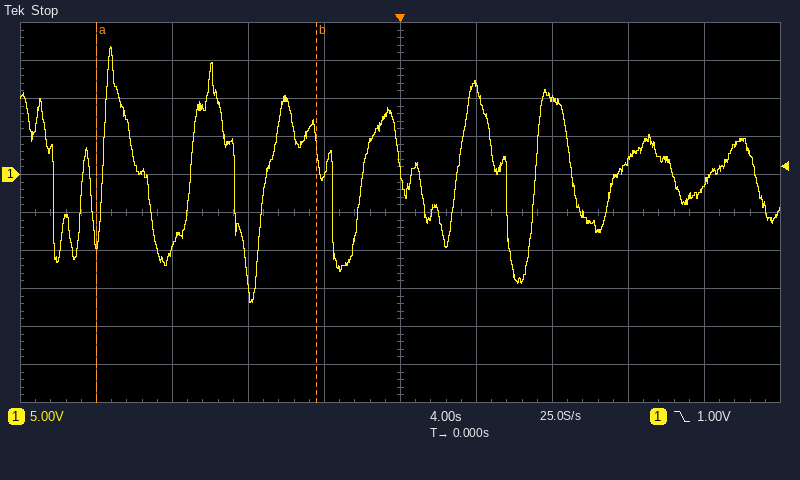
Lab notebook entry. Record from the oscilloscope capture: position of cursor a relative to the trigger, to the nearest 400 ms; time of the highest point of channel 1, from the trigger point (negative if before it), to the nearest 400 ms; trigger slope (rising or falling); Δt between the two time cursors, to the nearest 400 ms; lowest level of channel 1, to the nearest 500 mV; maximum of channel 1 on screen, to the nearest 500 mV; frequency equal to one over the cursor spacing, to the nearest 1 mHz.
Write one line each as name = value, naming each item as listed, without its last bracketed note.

position of cursor a relative to the trigger, to the nearest 400 ms = -16.0 s
time of the highest point of channel 1, from the trigger point (negative if before it), to the nearest 400 ms = -15.2 s
trigger slope = falling
Δt between the two time cursors, to the nearest 400 ms = 11.6 s
lowest level of channel 1, to the nearest 500 mV = -17.0 V
maximum of channel 1 on screen, to the nearest 500 mV = 17.0 V
frequency equal to one over the cursor spacing, to the nearest 1 mHz = 86 mHz
